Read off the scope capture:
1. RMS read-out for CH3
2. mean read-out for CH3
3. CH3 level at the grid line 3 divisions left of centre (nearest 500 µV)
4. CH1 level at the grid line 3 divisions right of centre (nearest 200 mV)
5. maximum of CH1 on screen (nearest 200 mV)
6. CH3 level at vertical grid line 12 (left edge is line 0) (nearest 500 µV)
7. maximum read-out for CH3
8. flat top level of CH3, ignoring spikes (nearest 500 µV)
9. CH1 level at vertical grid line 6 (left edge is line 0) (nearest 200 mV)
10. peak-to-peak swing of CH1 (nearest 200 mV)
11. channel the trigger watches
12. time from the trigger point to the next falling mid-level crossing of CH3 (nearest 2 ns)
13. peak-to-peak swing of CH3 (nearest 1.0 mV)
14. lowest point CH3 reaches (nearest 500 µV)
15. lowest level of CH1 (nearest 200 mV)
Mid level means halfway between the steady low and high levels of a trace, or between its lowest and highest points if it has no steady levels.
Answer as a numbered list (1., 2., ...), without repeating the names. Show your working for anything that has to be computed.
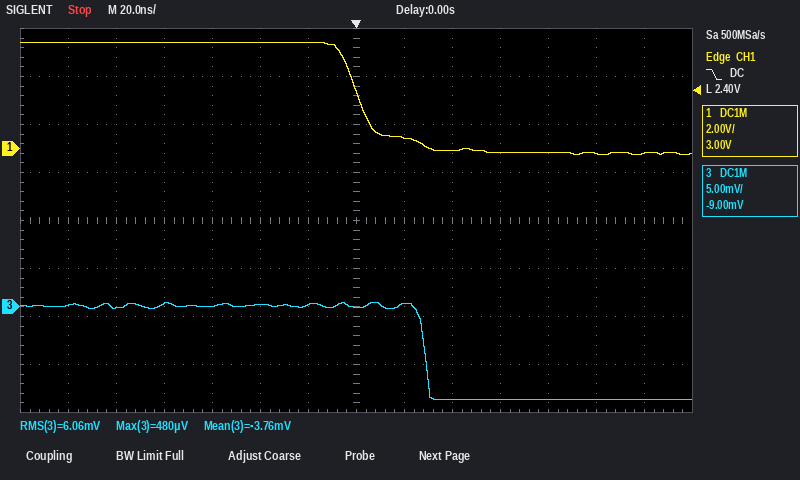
1. 6.06 mV
2. -3.76 mV
3. 0.0 mV
4. -200 mV
5. 4.4 V
6. -9.5 mV
7. 480 µV
8. 0.0 mV
9. 4.4 V
10. 4.4 V − (-200 mV) = 4.6 V
11. CH1
12. 28 ns
13. 10.0 mV
14. -9.5 mV
15. -200 mV
